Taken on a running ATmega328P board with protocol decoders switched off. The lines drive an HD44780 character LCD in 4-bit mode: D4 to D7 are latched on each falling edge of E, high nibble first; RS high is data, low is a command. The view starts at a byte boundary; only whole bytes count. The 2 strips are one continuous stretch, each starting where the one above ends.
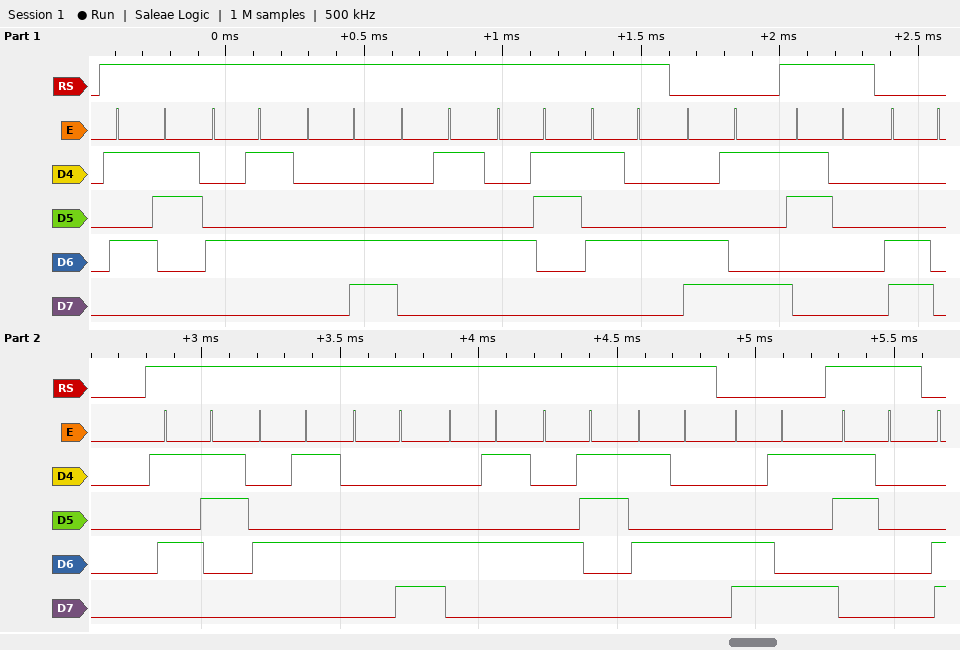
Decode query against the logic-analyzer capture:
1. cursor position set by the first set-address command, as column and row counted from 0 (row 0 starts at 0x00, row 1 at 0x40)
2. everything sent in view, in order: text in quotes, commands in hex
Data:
column 9, row 1
"SELECT" 0xC9 "0" 0xC0 "SELECT" 0xC9 "0"
